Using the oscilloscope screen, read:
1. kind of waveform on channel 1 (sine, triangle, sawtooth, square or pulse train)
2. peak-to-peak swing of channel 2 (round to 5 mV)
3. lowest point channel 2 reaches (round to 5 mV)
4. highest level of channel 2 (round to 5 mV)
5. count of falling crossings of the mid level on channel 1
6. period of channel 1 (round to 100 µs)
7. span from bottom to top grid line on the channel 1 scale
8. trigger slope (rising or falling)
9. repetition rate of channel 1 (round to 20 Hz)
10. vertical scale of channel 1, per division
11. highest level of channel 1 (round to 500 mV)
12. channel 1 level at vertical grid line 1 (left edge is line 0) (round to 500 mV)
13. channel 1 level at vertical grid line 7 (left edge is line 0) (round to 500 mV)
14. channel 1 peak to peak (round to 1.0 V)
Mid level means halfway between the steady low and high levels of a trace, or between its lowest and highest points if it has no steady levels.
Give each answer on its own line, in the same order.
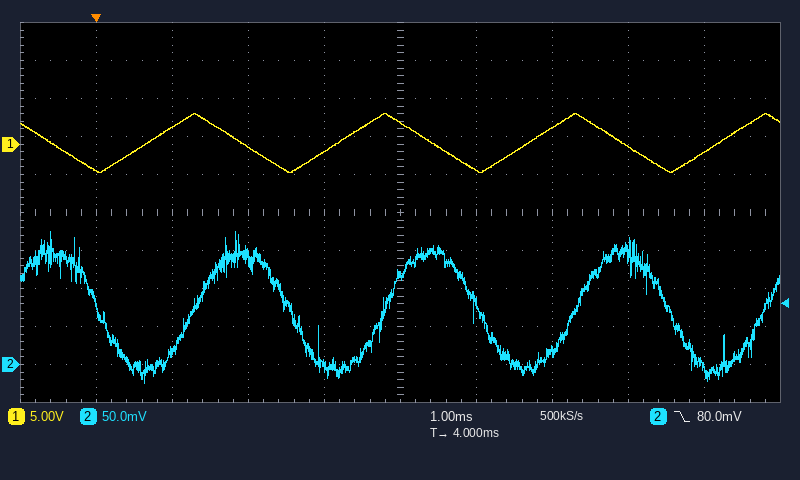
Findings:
triangle
200 mV
-25 mV
175 mV
4
2.5 ms
50 V
falling
400 Hz
5 V
4.0 V
-3.5 V
2.0 V
8.0 V
